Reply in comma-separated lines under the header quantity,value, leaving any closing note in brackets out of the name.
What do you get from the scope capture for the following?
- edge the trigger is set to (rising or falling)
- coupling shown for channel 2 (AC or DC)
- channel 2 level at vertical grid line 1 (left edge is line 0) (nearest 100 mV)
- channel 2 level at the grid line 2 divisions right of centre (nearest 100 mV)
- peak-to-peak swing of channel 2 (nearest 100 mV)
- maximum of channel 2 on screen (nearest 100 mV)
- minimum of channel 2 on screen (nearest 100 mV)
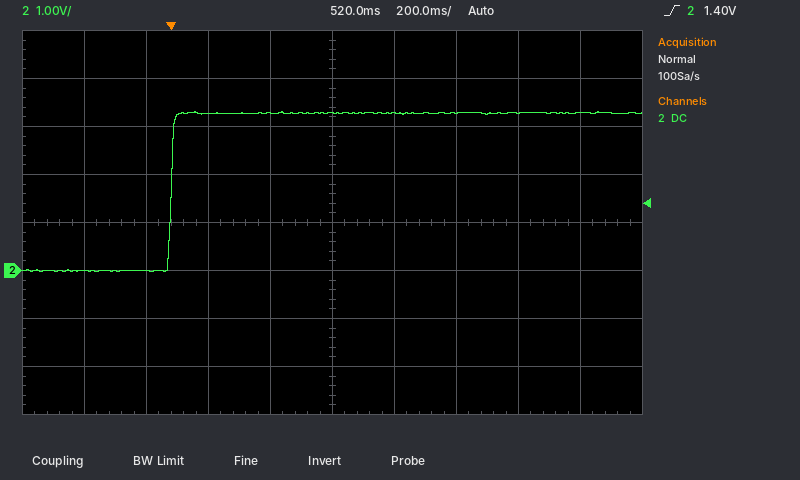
quantity,value
edge the trigger is set to,rising
coupling shown for channel 2,DC
channel 2 level at vertical grid line 1 (left edge is line 0),0.0 V
channel 2 level at the grid line 2 divisions right of centre,3.3 V
peak-to-peak swing of channel 2,3.3 V
maximum of channel 2 on screen,3.3 V
minimum of channel 2 on screen,0.0 V
